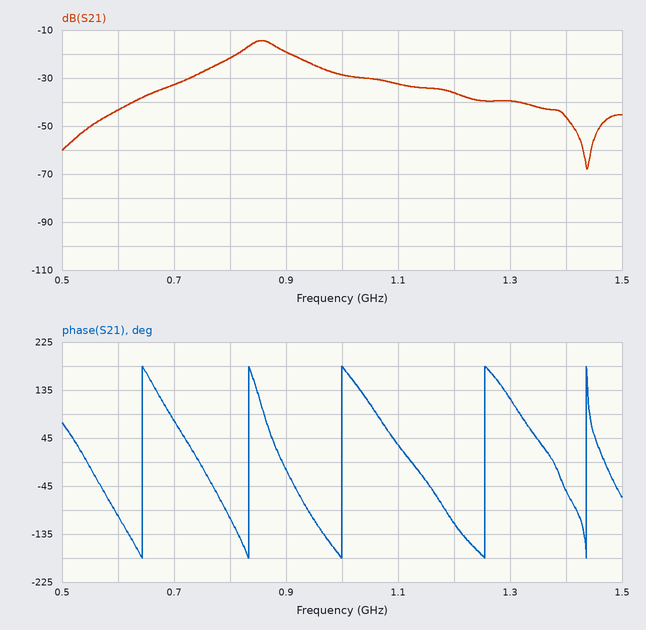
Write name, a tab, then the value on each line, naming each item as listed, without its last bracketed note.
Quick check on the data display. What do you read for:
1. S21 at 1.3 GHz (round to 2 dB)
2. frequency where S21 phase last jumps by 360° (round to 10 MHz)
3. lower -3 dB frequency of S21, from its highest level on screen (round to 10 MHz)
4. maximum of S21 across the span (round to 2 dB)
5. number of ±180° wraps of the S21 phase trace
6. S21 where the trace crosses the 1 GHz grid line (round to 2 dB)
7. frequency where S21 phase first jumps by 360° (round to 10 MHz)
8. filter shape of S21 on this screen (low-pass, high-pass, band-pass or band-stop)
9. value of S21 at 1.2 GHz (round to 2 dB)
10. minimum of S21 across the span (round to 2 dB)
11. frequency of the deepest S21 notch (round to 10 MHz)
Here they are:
S21 at 1.3 GHz	-40 dB
frequency where S21 phase last jumps by 360°	1.44 GHz
lower -3 dB frequency of S21, from its highest level on screen	830 MHz
maximum of S21 across the span	-14 dB
number of ±180° wraps of the S21 phase trace	5
S21 where the trace crosses the 1 GHz grid line	-28 dB
frequency where S21 phase first jumps by 360°	640 MHz
filter shape of S21 on this screen	band-pass
value of S21 at 1.2 GHz	-36 dB
minimum of S21 across the span	-68 dB
frequency of the deepest S21 notch	1.44 GHz
